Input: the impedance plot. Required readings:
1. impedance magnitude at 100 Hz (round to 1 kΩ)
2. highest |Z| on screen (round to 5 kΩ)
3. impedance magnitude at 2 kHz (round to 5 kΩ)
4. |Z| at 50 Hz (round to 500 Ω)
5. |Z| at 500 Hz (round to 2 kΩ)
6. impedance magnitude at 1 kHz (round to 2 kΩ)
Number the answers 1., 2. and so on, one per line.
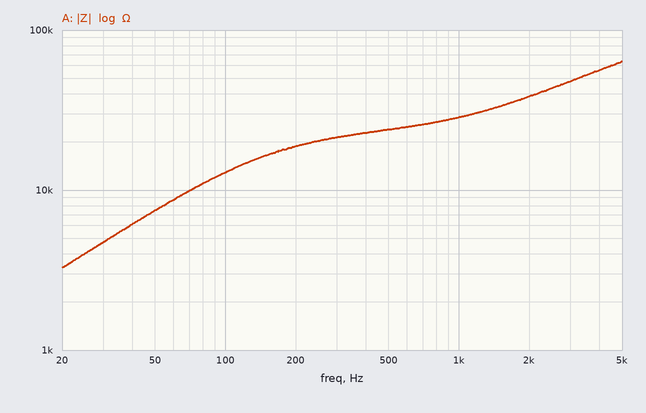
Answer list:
1. 13 kΩ
2. 65 kΩ
3. 40 kΩ
4. 7.5 kΩ
5. 24 kΩ
6. 28 kΩ
